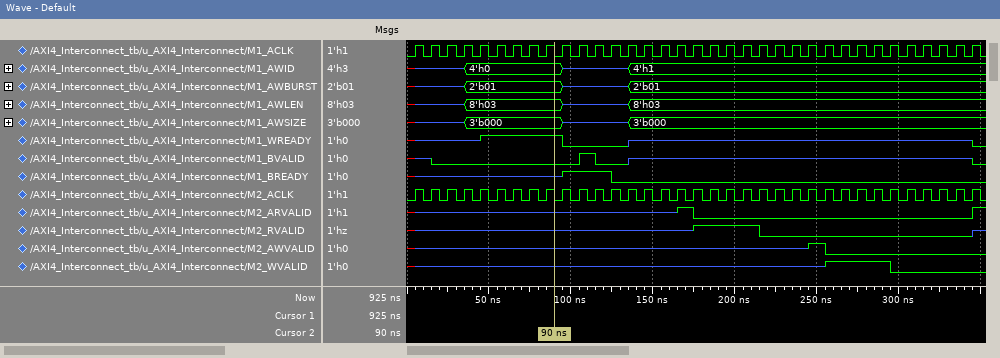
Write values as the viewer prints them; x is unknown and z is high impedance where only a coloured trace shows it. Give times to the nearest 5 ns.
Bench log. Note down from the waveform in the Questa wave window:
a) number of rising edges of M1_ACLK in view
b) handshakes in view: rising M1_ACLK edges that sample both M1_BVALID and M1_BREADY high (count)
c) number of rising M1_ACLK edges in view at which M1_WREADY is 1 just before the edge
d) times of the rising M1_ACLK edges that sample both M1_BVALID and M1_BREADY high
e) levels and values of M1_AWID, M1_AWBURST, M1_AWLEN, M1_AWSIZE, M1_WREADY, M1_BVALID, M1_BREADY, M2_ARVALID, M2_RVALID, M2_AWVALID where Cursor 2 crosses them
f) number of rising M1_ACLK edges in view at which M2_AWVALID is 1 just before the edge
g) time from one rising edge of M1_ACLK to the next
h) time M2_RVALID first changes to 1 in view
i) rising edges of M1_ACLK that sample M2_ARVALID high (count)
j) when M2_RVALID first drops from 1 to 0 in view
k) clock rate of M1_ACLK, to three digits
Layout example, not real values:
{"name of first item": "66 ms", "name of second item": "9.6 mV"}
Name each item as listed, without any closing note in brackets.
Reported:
{"number of rising edges of M1_ACLK in view": "35", "handshakes in view: rising M1_ACLK edges that sample both M1_BVALID and M1_BREADY high": "1", "number of rising M1_ACLK edges in view at which M1_WREADY is 1 just before the edge": "5", "times of the rising M1_ACLK edges that sample both M1_BVALID and M1_BREADY high": "115 ns", "levels and values of M1_AWID, M1_AWBURST, M1_AWLEN, M1_AWSIZE, M1_WREADY, M1_BVALID, M1_BREADY, M2_ARVALID, M2_RVALID, M2_AWVALID where Cursor 2 crosses them": "M1_AWID=4'h0, M1_AWBURST=2'b01, M1_AWLEN=8'h03, M1_AWSIZE=3'b000, M1_WREADY=1, M1_BVALID=0, M1_BREADY=z, M2_ARVALID=z, M2_RVALID=z, M2_AWVALID=z", "number of rising M1_ACLK edges in view at which M2_AWVALID is 1 just before the edge": "1", "time from one rising edge of M1_ACLK to the next": "10 ns", "time M2_RVALID first changes to 1 in view": "175 ns", "rising edges of M1_ACLK that sample M2_ARVALID high": "1", "when M2_RVALID first drops from 1 to 0 in view": "215 ns", "clock rate of M1_ACLK, to three digits": "100 MHz"}
